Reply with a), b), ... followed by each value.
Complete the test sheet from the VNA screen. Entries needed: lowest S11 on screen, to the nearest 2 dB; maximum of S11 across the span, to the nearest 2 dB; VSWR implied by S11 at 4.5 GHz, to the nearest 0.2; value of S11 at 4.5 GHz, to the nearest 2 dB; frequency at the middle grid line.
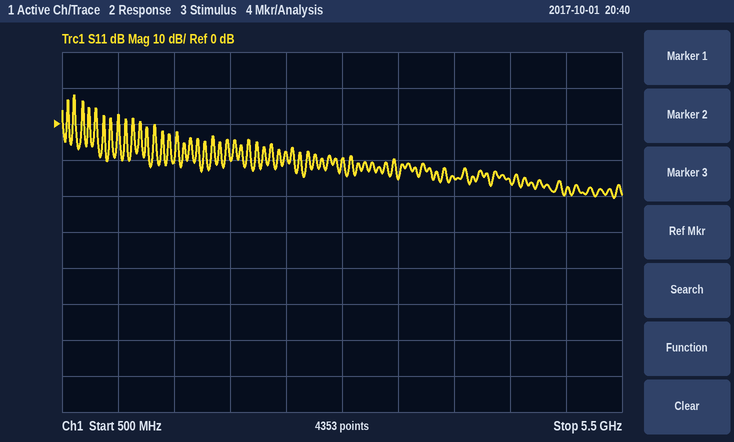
a) -20 dB
b) 8 dB
c) 1.4
d) -16 dB
e) 3 GHz
